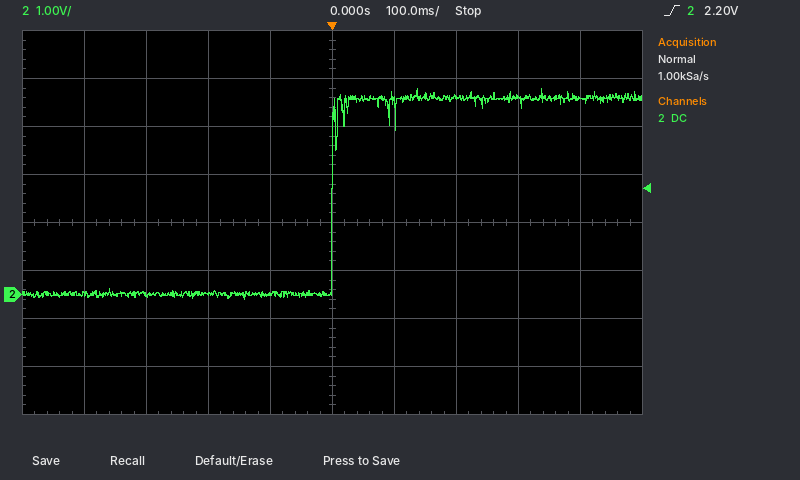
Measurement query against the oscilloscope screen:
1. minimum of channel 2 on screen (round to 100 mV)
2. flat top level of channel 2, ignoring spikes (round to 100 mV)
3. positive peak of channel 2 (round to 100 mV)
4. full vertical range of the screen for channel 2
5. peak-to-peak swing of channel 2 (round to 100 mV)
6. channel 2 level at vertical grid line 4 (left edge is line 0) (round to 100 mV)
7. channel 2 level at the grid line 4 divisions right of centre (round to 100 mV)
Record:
-100 mV
4.1 V
4.3 V
8 V
4.4 V
0.0 V
4.1 V
